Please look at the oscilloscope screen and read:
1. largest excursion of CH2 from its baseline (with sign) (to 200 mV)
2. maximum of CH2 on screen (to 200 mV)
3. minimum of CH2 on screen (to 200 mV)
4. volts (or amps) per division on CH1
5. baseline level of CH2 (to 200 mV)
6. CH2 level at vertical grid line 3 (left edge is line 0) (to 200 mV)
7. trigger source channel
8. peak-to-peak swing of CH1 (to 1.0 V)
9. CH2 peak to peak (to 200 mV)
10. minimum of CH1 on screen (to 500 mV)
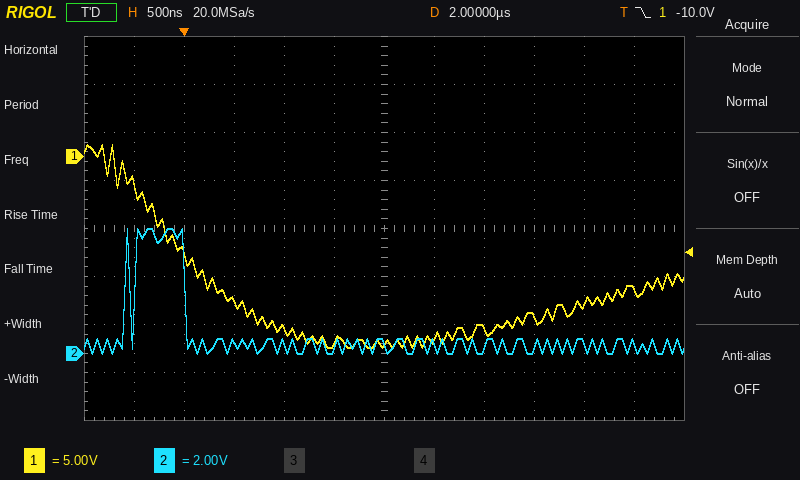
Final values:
+4.8 V
5.2 V
0.0 V
5 V
400 mV
400 mV
CH1
21.0 V
5.2 V
-20.0 V
